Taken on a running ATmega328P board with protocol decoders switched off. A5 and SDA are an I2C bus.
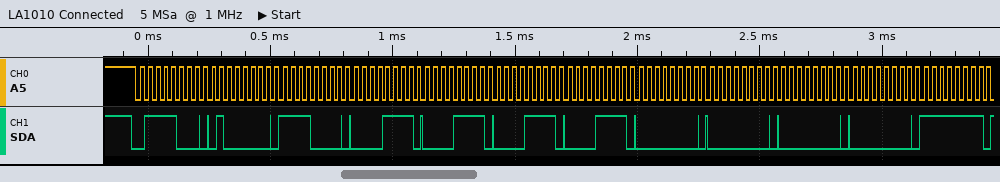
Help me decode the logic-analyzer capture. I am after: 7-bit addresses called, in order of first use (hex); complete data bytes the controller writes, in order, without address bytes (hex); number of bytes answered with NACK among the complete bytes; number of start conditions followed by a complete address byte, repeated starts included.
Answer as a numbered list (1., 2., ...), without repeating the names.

1. 0x3C
2. 40 F0 0F 0F 0F 0F 00 00 00 00 FF
3. 0
4. 1
